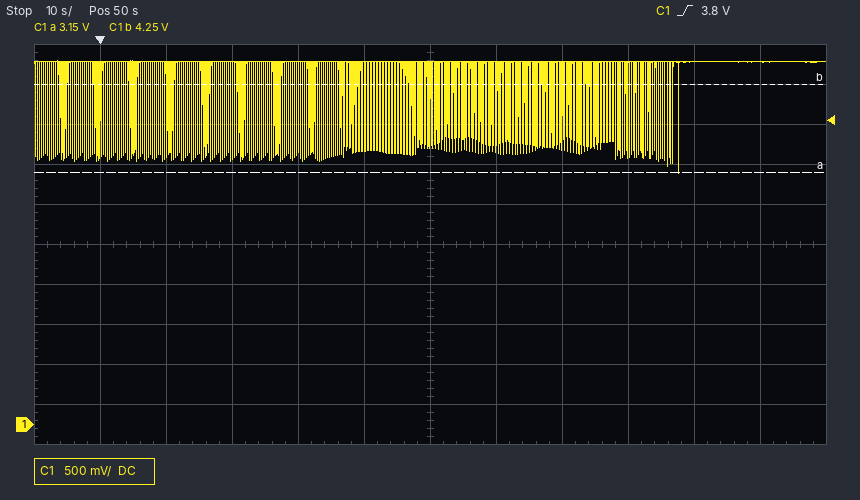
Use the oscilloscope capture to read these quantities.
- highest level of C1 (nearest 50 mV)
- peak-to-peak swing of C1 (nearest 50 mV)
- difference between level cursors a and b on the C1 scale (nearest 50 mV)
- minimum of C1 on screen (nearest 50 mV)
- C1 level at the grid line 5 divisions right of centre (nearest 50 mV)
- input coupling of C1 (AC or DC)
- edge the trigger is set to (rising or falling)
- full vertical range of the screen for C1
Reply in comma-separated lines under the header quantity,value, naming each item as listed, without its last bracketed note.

quantity,value
highest level of C1,4.55 V
peak-to-peak swing of C1,1.40 V
difference between level cursors a and b on the C1 scale,1.10 V
minimum of C1 on screen,3.15 V
C1 level at the grid line 5 divisions right of centre,4.55 V
input coupling of C1,DC
edge the trigger is set to,rising
full vertical range of the screen for C1,5 V
